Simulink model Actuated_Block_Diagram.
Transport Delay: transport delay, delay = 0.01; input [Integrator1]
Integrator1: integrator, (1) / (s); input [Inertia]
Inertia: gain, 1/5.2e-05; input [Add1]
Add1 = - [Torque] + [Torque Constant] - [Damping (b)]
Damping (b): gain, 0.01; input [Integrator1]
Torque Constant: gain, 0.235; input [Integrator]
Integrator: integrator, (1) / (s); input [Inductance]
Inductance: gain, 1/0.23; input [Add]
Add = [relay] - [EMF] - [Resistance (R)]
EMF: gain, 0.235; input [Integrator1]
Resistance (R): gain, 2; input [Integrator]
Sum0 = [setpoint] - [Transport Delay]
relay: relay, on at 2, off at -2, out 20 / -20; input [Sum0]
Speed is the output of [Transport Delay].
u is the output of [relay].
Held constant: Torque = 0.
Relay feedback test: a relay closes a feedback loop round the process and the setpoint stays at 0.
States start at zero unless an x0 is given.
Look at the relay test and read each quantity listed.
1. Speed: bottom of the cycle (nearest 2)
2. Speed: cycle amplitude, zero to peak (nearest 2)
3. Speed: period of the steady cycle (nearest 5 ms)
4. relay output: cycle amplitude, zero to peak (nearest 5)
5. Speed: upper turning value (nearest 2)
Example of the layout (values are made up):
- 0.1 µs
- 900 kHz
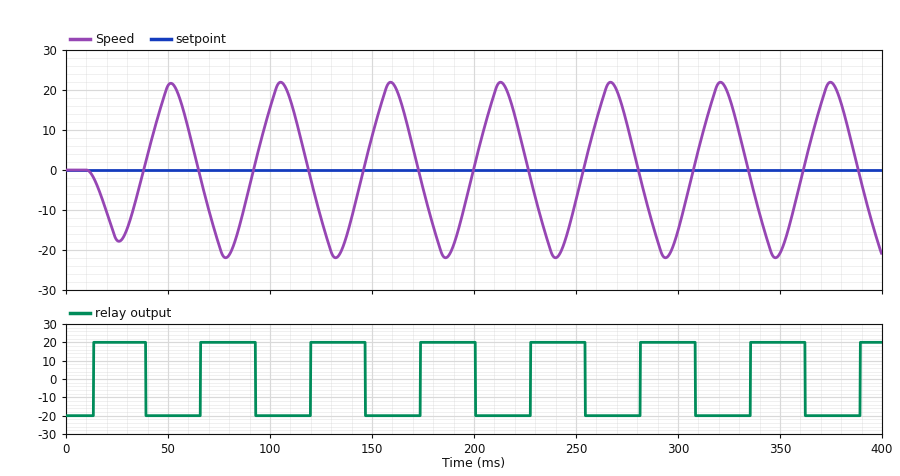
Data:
- -22
- 22
- 55 ms
- 20
- 22
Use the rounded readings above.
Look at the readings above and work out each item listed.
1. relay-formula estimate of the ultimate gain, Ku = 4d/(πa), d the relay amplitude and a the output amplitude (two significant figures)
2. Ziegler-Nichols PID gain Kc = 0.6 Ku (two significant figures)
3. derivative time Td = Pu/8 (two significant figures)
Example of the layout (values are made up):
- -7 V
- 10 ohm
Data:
- 1.2
- 0.72
- 6.9 ms
